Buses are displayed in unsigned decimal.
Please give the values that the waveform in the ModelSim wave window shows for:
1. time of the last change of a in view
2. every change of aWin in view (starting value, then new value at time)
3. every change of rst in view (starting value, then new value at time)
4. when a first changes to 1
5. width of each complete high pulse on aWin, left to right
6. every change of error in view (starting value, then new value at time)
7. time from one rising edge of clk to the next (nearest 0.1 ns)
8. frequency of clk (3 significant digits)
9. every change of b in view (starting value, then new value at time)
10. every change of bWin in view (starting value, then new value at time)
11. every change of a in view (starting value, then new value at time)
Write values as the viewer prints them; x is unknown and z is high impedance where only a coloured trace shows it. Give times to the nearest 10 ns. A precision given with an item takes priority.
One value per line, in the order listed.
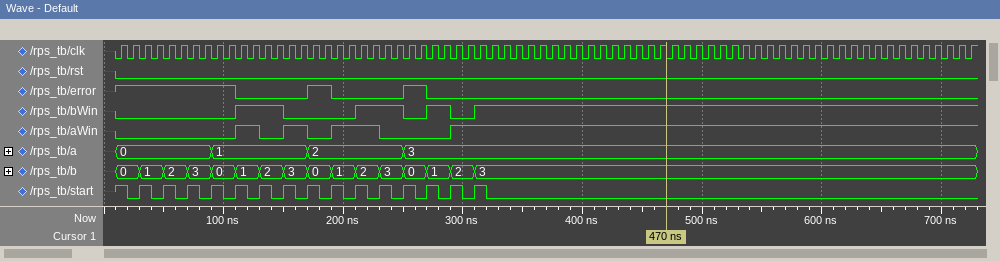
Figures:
250 ns
x, 0 at 10 ns, 1 at 110 ns, 0 at 130 ns, 1 at 150 ns, 0 at 170 ns, 1 at 190 ns, 0 at 230 ns, 1 at 290 ns
x, 0 at 10 ns
90 ns
20 ns, 20 ns, 40 ns
x, 1 at 10 ns, 0 at 110 ns, 1 at 170 ns, 0 at 190 ns, 1 at 250 ns, 0 at 270 ns
10 ns
100 MHz
x, 0 at 10 ns, 1 at 30 ns, 2 at 50 ns, 3 at 70 ns, 0 at 90 ns, 1 at 110 ns, 2 at 130 ns, 3 at 150 ns, 0 at 170 ns, 1 at 190 ns, 2 at 210 ns, 3 at 230 ns, 0 at 250 ns, 1 at 270 ns, 2 at 290 ns, 3 at 310 ns
x, 0 at 10 ns, 1 at 110 ns, 0 at 150 ns, 1 at 210 ns, 0 at 250 ns, 1 at 270 ns, 0 at 290 ns, 1 at 310 ns
x, 0 at 10 ns, 1 at 90 ns, 2 at 170 ns, 3 at 250 ns
